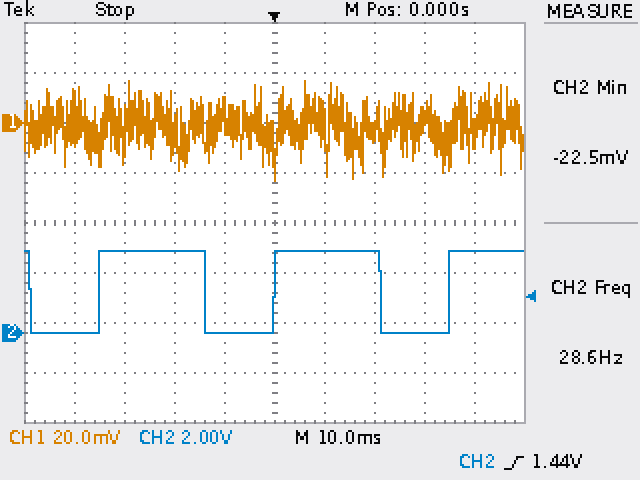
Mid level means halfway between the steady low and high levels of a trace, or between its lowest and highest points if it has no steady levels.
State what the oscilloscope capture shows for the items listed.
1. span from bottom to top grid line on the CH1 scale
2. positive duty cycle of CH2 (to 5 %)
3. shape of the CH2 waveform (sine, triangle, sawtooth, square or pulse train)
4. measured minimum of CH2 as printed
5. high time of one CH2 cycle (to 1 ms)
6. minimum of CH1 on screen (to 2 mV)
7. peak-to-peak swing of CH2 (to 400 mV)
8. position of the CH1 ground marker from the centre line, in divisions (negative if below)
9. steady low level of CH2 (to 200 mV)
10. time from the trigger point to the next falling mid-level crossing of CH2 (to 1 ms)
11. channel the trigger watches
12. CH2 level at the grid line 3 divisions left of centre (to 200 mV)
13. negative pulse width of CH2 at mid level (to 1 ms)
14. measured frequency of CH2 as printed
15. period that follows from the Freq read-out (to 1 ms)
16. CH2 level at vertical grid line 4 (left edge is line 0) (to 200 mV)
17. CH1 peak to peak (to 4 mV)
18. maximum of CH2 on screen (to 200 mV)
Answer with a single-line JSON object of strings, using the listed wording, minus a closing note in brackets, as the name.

{"span from bottom to top grid line on the CH1 scale": "160 mV", "positive duty cycle of CH2": "60 %", "shape of the CH2 waveform": "pulse train", "measured minimum of CH2 as printed": "-22.5 mV", "high time of one CH2 cycle": "21 ms", "minimum of CH1 on screen": "-24 mV", "peak-to-peak swing of CH2": "3.2 V", "position of the CH1 ground marker from the centre line, in divisions": "+2.0 div", "steady low level of CH2": "0.0 V", "time from the trigger point to the next falling mid-level crossing of CH2": "21 ms", "channel the trigger watches": "CH2", "CH2 level at the grid line 3 divisions left of centre": "3.2 V", "negative pulse width of CH2 at mid level": "14 ms", "measured frequency of CH2 as printed": "28.6 Hz", "period that follows from the Freq read-out": "35 ms", "CH2 level at vertical grid line 4 (left edge is line 0)": "0.0 V", "CH1 peak to peak": "40 mV", "maximum of CH2 on screen": "3.2 V"}
